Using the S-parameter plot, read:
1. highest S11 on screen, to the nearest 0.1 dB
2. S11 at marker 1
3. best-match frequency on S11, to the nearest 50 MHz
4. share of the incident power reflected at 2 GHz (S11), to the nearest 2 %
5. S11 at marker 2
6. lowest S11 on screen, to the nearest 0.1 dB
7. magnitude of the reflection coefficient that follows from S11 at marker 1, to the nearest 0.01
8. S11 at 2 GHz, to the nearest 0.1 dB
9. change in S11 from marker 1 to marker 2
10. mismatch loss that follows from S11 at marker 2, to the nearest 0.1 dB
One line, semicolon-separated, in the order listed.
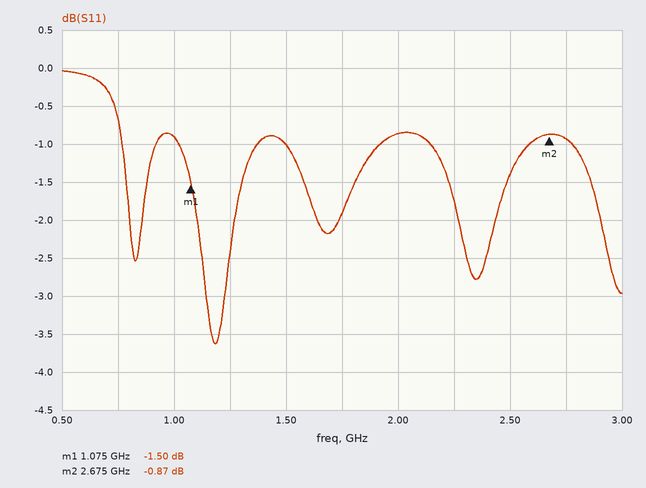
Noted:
0.0 dB; -1.50 dB; 1.20 GHz; 82 %; -0.87 dB; -3.6 dB; 0.84; -0.9 dB; 0.63 dB; 7.4 dB
